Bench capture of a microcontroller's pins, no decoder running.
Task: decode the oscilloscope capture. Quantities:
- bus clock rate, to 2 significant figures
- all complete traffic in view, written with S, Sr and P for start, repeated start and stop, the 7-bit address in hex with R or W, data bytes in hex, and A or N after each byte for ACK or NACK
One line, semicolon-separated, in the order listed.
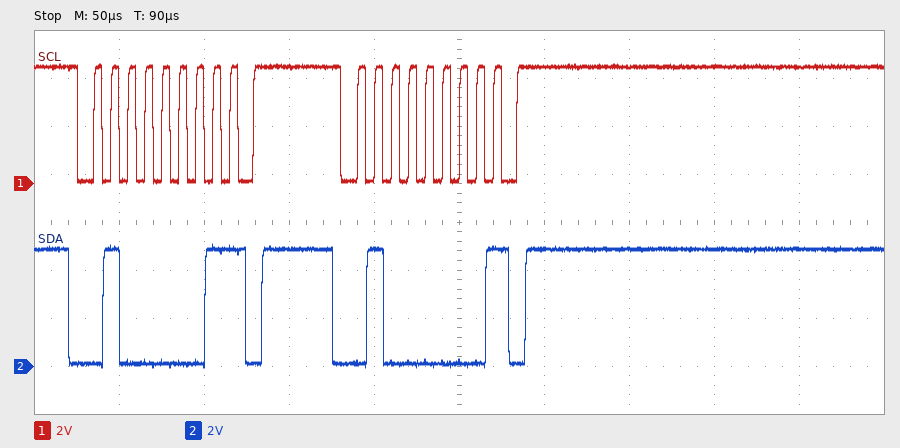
100 kHz; S 20R N P S 20W N P
